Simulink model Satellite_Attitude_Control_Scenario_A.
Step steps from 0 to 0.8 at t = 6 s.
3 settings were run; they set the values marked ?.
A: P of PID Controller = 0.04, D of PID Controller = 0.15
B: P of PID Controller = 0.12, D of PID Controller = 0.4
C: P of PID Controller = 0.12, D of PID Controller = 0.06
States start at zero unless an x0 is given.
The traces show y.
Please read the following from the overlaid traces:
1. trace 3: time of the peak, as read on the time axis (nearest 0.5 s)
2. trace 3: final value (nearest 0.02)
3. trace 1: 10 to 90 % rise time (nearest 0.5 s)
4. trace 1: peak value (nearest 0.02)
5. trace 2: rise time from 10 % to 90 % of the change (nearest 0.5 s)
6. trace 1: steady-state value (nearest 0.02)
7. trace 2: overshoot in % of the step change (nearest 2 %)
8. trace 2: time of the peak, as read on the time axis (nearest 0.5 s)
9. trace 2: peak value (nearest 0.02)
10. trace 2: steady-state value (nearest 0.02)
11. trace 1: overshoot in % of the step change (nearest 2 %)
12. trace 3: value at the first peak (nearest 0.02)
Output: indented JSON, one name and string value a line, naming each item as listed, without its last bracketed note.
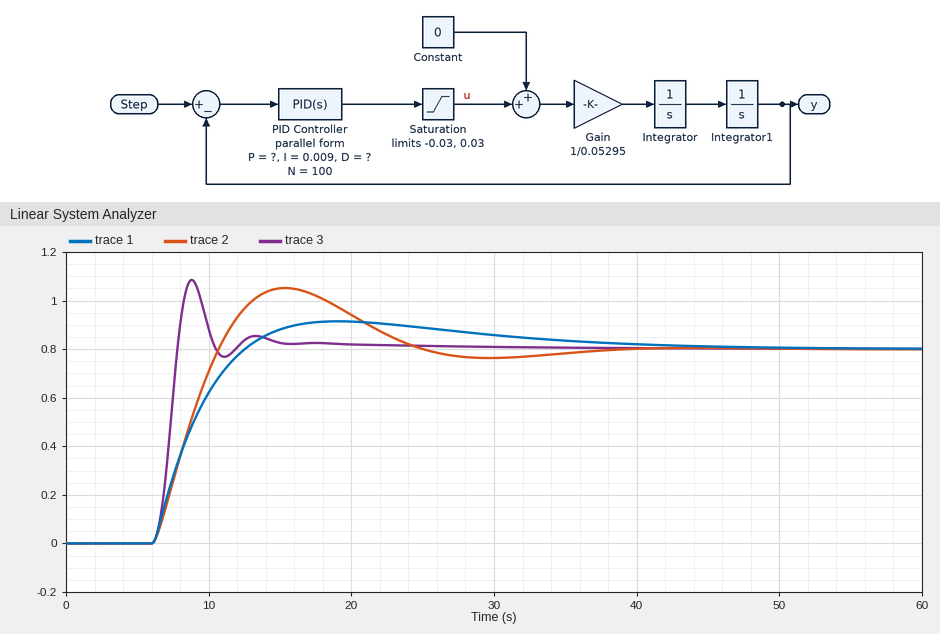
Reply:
{
  "trace 3: time of the peak, as read on the time axis": "9.0 s",
  "trace 3: final value": "0.80",
  "trace 1: 10 to 90 % rise time": "4.5 s",
  "trace 1: peak value": "0.92",
  "trace 2: rise time from 10 % to 90 % of the change": "3.5 s",
  "trace 1: steady-state value": "0.80",
  "trace 2: overshoot in % of the step change": "32 %",
  "trace 2: time of the peak, as read on the time axis": "15.5 s",
  "trace 2: peak value": "1.06",
  "trace 2: steady-state value": "0.80",
  "trace 1: overshoot in % of the step change": "14 %",
  "trace 3: value at the first peak": "1.08"
}
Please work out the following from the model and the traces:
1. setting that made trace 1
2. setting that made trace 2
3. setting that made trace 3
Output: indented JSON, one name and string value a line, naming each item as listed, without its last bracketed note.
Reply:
{
  "setting that made trace 1": "B",
  "setting that made trace 2": "A",
  "setting that made trace 3": "C"
}
